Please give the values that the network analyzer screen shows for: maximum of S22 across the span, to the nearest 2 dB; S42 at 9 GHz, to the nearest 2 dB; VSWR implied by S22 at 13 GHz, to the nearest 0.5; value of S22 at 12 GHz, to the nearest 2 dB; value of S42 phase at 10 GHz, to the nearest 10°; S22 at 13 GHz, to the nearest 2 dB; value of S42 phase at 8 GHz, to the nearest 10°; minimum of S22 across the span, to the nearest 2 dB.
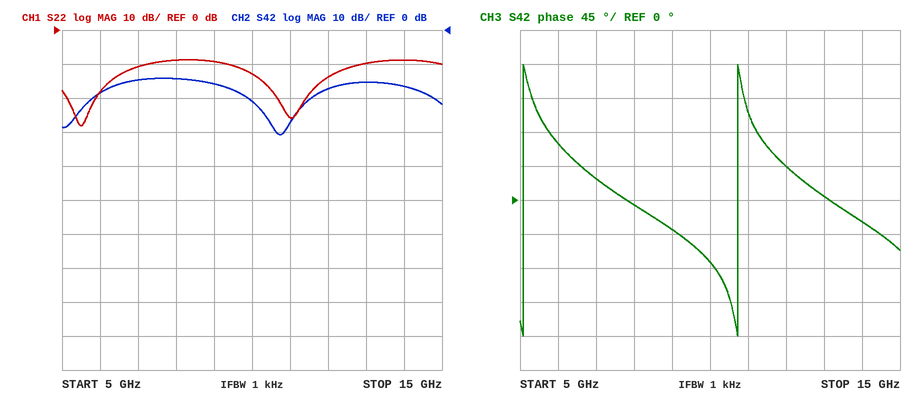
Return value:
-8 dB
-16 dB
2.0
-14 dB
-80°
-10 dB
-10°
-28 dB
